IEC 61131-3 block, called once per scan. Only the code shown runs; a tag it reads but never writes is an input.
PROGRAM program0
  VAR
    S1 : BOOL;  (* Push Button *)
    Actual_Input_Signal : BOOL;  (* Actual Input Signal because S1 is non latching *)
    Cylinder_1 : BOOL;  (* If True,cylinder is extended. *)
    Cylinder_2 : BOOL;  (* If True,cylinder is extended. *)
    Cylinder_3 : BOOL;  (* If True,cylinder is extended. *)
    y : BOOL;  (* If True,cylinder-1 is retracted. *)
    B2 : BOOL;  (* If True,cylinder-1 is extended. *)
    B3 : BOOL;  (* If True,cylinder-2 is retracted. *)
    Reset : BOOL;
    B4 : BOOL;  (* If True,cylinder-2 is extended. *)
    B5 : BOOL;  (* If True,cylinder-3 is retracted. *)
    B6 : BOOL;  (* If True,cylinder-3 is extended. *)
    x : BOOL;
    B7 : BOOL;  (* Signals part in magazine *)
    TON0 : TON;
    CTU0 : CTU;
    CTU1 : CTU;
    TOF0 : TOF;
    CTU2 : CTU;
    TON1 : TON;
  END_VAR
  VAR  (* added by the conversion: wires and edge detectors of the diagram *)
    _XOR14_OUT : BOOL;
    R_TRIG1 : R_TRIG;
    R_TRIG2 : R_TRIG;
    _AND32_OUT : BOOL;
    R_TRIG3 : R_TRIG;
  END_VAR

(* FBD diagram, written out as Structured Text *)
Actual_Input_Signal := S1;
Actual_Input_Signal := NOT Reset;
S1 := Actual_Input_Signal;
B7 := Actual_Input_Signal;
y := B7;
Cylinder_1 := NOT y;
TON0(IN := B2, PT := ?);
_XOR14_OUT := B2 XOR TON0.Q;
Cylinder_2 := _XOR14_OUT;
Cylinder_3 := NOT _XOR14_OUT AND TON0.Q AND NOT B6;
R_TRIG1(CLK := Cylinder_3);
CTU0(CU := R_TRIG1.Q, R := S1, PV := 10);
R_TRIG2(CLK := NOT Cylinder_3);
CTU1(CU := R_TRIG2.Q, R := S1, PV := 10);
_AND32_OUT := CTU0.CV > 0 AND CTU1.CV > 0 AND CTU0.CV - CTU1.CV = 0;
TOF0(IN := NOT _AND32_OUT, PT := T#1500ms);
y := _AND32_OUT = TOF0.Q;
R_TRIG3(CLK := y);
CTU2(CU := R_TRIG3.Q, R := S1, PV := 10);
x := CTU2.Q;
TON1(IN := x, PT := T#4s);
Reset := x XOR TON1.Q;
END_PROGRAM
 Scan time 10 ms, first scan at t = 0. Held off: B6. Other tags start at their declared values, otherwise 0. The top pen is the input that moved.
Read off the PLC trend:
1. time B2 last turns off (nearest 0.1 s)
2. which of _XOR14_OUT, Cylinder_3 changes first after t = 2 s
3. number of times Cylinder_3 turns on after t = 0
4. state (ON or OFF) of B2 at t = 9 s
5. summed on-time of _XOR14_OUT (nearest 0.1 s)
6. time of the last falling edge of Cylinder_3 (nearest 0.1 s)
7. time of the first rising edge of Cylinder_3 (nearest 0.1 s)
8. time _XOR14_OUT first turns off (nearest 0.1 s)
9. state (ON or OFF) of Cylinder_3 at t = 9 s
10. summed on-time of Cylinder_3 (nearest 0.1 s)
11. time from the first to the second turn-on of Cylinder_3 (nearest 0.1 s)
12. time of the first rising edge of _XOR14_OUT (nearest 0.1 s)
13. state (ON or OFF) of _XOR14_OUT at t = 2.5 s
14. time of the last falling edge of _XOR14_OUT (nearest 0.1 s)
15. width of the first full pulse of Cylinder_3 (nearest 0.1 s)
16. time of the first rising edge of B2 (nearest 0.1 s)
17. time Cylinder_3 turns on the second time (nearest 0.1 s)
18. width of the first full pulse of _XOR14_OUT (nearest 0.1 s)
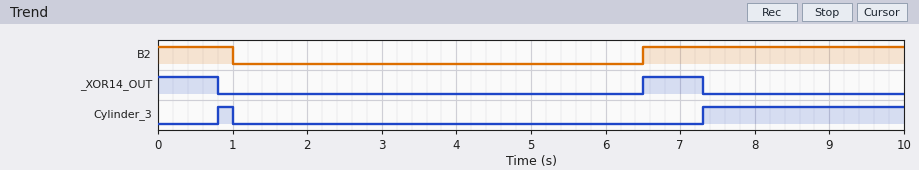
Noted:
1.0 s
_XOR14_OUT
2
ON
1.6 s
1.0 s
0.8 s
0.8 s
ON
2.9 s
6.5 s
6.5 s
OFF
7.3 s
0.2 s
6.5 s
7.3 s
0.8 s
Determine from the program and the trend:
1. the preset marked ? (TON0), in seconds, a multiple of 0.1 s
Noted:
0.8 s
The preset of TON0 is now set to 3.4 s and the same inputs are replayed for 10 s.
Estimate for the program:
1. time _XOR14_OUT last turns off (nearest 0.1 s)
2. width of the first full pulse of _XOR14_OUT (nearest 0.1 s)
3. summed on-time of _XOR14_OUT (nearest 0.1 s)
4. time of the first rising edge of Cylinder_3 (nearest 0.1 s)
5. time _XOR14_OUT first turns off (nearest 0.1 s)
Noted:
9.9 s
3.4 s
4.4 s
9.9 s
1.0 s
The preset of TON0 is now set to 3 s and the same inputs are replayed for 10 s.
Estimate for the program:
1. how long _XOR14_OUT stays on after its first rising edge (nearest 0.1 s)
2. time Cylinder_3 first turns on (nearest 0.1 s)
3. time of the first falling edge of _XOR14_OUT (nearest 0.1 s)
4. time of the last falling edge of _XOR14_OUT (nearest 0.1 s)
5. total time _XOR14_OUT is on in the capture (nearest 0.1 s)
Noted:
3.0 s
9.5 s
1.0 s
9.5 s
4.0 s
